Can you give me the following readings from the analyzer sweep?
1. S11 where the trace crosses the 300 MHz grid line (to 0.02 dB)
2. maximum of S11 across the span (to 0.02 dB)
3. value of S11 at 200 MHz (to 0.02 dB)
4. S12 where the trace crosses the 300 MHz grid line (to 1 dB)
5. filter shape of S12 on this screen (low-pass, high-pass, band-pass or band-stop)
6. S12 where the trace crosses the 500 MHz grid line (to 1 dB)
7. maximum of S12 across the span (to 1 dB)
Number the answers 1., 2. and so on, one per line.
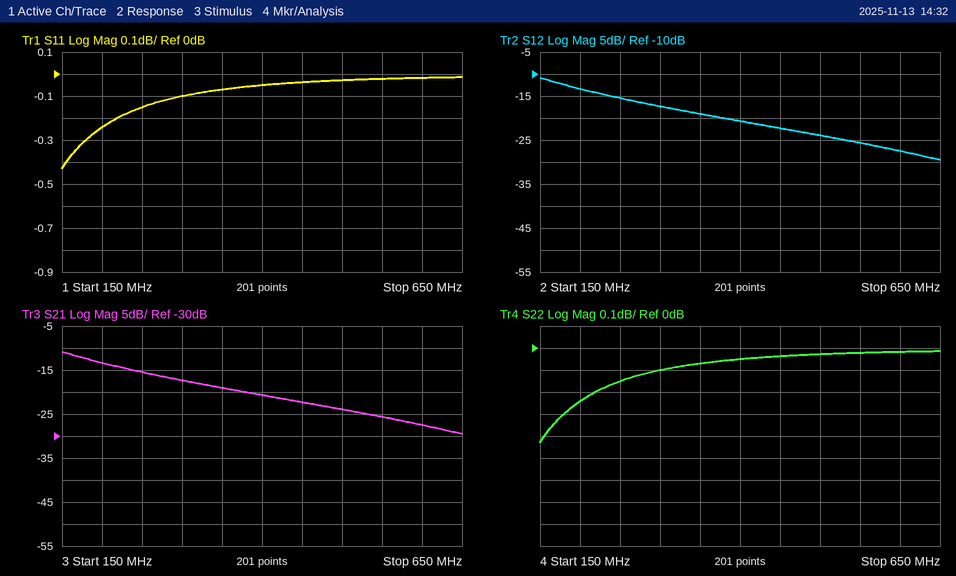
1. -0.10 dB
2. -0.02 dB
3. -0.24 dB
4. -17 dB
5. low-pass
6. -24 dB
7. -11 dB
